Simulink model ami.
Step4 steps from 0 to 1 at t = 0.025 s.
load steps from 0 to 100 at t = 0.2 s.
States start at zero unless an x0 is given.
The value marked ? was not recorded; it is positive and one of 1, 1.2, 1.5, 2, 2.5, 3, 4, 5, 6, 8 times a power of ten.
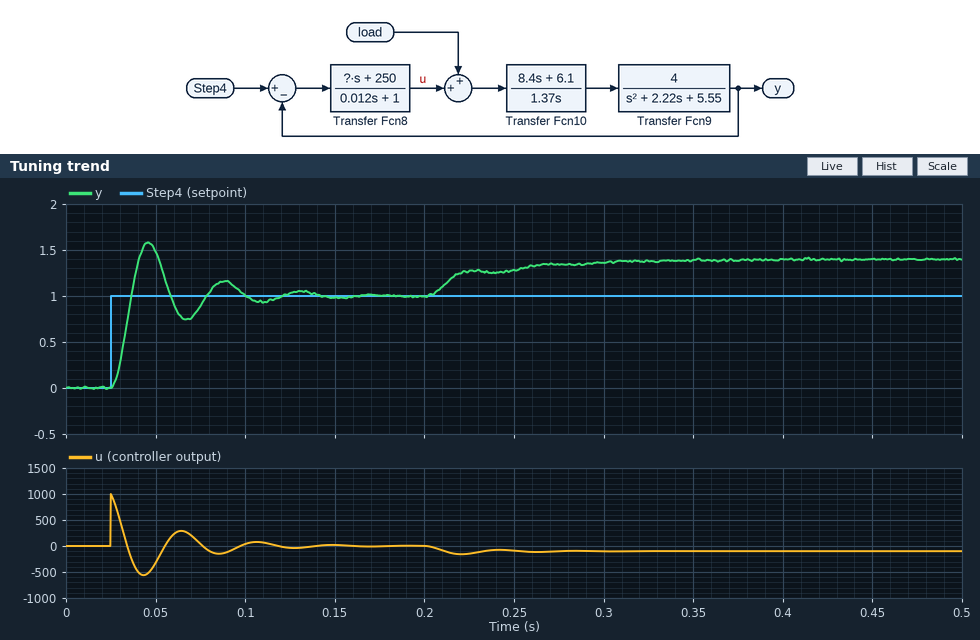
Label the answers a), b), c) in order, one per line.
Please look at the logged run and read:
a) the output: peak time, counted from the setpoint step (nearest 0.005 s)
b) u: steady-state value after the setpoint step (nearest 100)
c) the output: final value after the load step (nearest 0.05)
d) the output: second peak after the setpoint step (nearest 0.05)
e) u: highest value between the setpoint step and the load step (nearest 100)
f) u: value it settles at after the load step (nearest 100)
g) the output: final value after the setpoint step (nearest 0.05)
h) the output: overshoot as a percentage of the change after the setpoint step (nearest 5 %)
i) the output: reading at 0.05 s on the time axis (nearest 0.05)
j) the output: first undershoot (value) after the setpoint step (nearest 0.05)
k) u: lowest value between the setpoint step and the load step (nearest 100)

a) 0.020 s
b) 0
c) 1.40
d) 1.15
e) 1000
f) -100
g) 1.00
h) 60 %
i) 1.50
j) 0.75
k) -600
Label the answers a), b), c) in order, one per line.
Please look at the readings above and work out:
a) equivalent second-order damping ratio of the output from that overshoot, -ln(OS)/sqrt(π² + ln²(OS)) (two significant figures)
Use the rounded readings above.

a) 0.16
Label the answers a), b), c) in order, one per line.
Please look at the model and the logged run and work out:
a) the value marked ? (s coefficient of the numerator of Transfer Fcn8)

a) 12
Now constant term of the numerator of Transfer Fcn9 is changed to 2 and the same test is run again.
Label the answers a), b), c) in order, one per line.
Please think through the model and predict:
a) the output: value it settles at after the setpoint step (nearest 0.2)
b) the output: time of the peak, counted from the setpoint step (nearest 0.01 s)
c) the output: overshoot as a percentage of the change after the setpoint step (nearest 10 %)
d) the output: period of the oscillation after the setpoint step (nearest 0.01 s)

a) 1.0
b) 0.03 s
c) 50 %
d) 0.06 s
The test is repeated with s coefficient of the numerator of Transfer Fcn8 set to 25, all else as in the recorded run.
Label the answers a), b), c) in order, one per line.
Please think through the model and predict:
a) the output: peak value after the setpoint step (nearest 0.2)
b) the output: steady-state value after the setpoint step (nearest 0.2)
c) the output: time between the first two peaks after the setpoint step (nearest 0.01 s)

a) 1.6
b) 1.0
c) 0.03 s
